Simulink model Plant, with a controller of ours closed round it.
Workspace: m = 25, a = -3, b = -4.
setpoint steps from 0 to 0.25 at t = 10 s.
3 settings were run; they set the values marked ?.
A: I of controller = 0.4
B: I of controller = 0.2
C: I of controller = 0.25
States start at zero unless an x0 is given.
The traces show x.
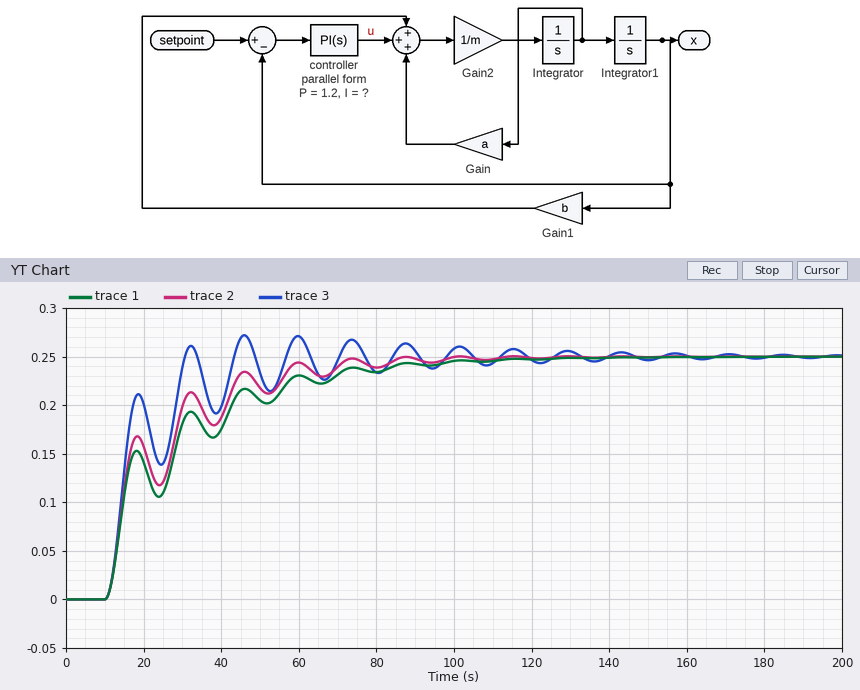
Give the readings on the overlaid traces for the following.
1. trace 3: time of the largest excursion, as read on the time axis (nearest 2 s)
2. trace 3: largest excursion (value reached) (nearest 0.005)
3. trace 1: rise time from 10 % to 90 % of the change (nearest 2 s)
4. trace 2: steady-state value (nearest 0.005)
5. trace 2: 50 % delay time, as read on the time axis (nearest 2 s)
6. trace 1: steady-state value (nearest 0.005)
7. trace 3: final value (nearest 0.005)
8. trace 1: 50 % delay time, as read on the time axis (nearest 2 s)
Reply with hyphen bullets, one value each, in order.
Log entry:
- 46 s
- 0.270
- 46 s
- 0.250
- 16 s
- 0.250
- 0.250
- 16 s
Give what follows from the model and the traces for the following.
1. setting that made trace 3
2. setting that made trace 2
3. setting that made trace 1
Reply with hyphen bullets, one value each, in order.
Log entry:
- A
- C
- B
